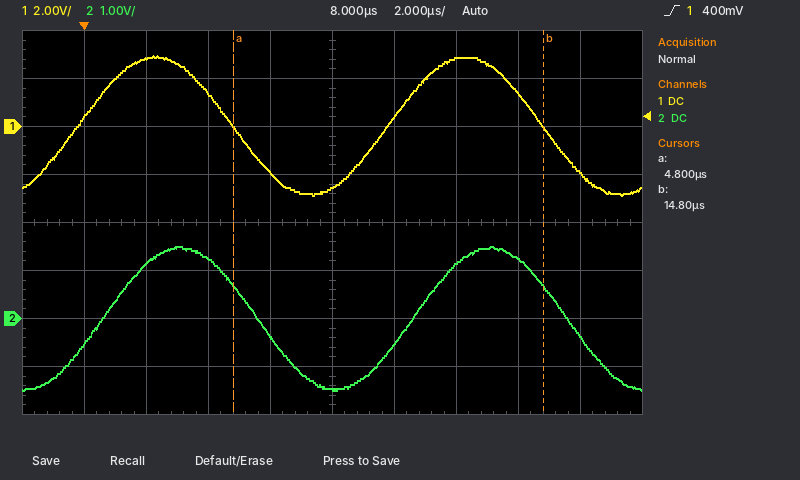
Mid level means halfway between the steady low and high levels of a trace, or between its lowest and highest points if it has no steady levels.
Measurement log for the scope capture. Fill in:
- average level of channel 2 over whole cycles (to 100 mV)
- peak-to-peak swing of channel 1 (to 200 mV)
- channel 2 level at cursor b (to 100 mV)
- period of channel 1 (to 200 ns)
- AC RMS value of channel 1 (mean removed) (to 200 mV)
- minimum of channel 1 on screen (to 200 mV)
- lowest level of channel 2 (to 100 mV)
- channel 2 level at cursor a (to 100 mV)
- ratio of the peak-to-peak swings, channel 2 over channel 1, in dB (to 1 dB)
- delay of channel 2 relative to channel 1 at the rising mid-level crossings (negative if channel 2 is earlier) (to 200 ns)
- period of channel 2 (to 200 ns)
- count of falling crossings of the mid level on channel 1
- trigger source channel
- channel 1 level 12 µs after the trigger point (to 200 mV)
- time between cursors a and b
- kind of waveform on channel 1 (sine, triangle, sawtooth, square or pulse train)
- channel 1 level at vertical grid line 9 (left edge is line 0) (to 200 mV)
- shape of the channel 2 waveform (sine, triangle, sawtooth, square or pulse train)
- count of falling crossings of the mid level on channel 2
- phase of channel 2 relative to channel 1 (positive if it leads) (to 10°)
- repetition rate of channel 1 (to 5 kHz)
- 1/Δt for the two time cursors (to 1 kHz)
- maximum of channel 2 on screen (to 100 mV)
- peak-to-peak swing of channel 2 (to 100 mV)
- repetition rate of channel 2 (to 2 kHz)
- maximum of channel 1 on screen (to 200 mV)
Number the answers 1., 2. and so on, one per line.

1. 0.0 V
2. 5.8 V
3. 700 mV
4. 10.0 µs
5. 2.0 V
6. -2.8 V
7. -1.5 V
8. 700 mV
9. -6 dB
10. +800 ns
11. 10.0 µs
12. 2
13. channel 1
14. 2.8 V
15. 10.0 µs
16. sine
17. -2.0 V
18. sine
19. 2
20. -30°
21. 100 kHz
22. 100 kHz
23. 1.5 V
24. 3.0 V
25. 100 kHz
26. 3.0 V
